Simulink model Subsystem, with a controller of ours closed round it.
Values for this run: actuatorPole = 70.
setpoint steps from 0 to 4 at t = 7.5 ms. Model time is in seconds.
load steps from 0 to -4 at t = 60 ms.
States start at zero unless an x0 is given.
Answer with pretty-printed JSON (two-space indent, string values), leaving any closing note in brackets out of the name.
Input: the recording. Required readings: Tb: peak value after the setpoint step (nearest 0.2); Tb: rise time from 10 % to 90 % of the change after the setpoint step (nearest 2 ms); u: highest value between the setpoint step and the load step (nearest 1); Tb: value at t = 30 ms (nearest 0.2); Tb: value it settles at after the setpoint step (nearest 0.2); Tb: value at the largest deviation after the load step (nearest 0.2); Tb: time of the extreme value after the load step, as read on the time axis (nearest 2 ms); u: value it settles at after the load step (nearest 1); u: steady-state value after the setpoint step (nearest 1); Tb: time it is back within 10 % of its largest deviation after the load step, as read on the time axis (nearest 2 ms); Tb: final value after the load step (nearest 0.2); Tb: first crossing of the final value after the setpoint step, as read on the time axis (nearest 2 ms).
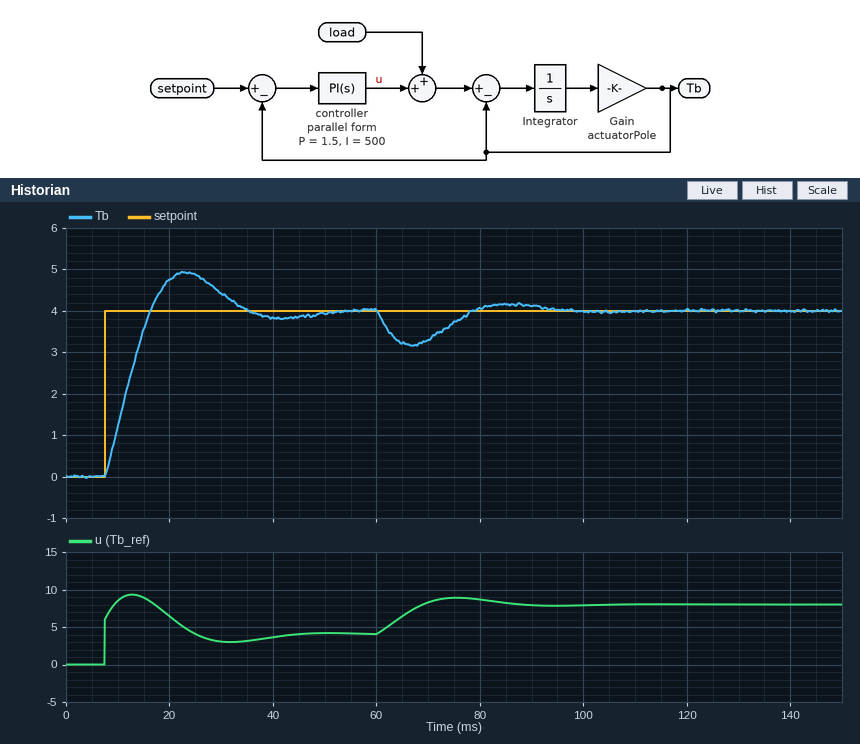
{
  "Tb: peak value after the setpoint step": "5.0",
  "Tb: rise time from 10 % to 90 % of the change after the setpoint step": "6 ms",
  "u: highest value between the setpoint step and the load step": "9",
  "Tb: value at t = 30 ms": "4.4",
  "Tb: value it settles at after the setpoint step": "4.0",
  "Tb: value at the largest deviation after the load step": "3.2",
  "Tb: time of the extreme value after the load step, as read on the time axis": "66 ms",
  "u: value it settles at after the load step": "8",
  "u: steady-state value after the setpoint step": "4",
  "Tb: time it is back within 10 % of its largest deviation after the load step, as read on the time axis": "92 ms",
  "Tb: final value after the load step": "4.0",
  "Tb: first crossing of the final value after the setpoint step, as read on the time axis": "16 ms"
}
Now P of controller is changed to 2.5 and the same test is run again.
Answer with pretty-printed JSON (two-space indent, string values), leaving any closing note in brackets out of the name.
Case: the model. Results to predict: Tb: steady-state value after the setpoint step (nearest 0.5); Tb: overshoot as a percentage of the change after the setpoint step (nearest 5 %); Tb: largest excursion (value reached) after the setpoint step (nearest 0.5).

{
  "Tb: steady-state value after the setpoint step": "4.0",
  "Tb: overshoot as a percentage of the change after the setpoint step": "15 %",
  "Tb: largest excursion (value reached) after the setpoint step": "4.5"
}
